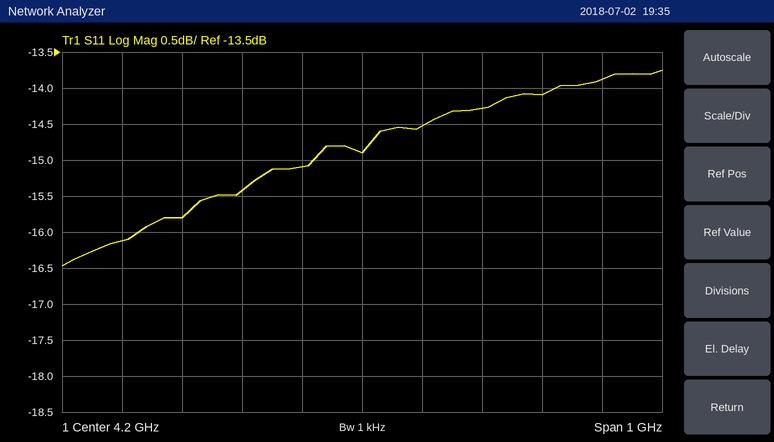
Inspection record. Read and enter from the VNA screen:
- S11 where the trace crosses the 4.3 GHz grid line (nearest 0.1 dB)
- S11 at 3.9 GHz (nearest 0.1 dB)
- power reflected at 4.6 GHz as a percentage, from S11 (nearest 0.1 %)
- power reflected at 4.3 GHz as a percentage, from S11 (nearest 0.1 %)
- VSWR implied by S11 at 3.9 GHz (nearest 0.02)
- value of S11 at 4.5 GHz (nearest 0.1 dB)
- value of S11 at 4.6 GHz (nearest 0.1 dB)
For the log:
-14.5 dB
-15.8 dB
4.1 %
3.5 %
1.38
-14.1 dB
-13.9 dB
